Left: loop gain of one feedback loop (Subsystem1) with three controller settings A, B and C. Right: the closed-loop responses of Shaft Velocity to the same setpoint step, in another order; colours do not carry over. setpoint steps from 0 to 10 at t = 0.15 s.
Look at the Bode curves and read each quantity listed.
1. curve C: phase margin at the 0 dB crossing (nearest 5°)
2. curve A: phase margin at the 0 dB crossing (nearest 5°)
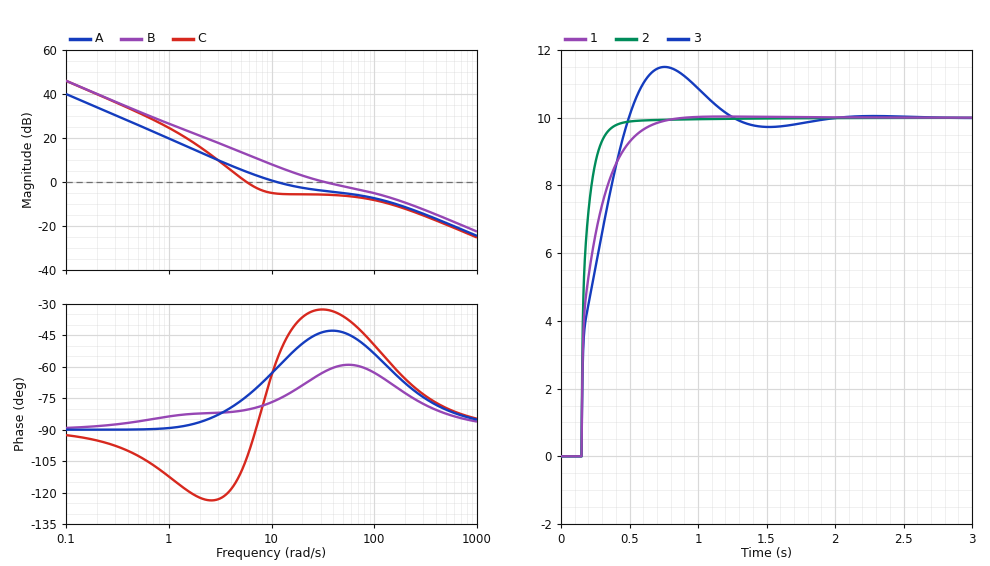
75°
120°
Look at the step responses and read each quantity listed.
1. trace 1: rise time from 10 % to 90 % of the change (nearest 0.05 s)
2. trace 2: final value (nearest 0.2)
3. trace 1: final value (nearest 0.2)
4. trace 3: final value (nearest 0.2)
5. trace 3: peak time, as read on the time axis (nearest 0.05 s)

0.30 s
10.0
10.0
10.0
0.75 s
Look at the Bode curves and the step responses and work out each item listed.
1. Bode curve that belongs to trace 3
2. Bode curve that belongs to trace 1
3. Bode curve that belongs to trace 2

C
A
B
